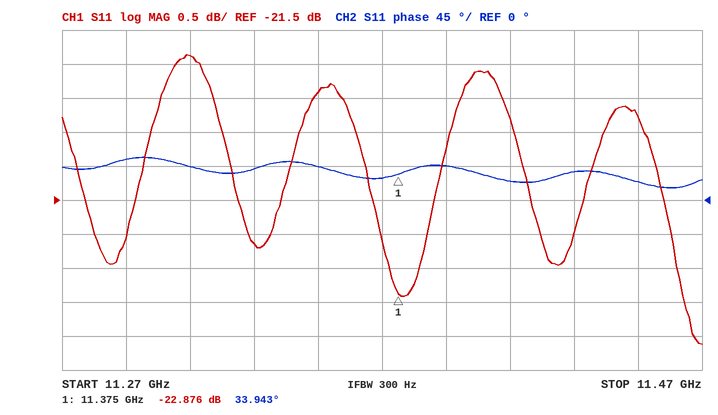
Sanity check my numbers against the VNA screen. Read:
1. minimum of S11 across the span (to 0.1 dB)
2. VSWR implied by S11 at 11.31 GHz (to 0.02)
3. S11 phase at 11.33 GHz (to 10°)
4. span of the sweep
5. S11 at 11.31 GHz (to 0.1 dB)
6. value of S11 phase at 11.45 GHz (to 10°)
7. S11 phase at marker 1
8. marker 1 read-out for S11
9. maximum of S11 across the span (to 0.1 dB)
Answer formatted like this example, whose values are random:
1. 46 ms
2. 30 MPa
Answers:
1. -23.6 dB
2. 1.24
3. 40°
4. 200 MHz
5. -19.4 dB
6. 20°
7. 33.943°
8. -22.876 dB
9. -19.4 dB
